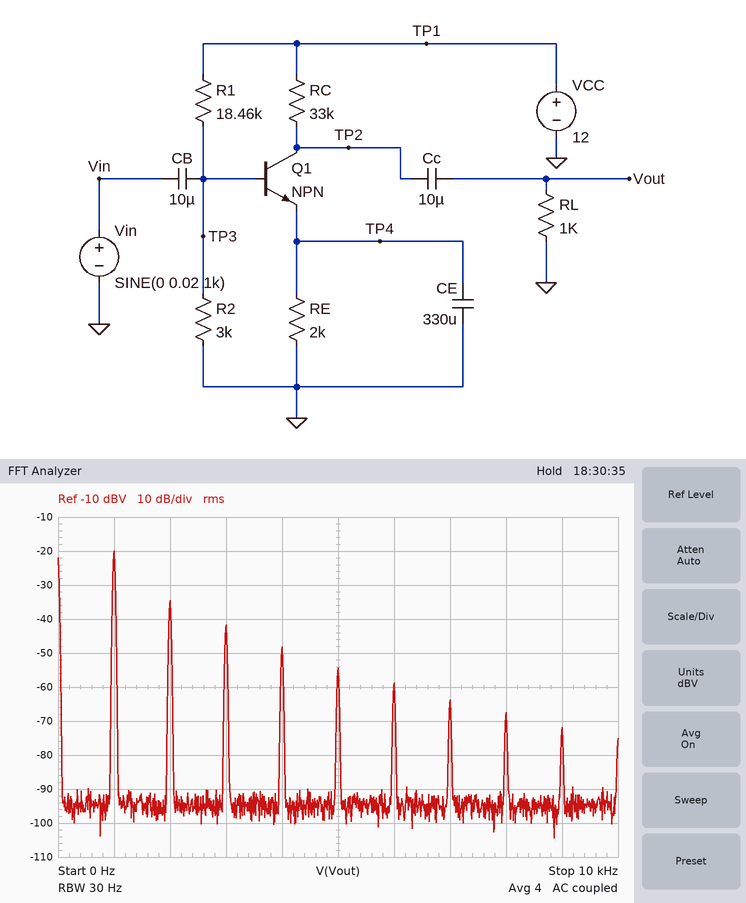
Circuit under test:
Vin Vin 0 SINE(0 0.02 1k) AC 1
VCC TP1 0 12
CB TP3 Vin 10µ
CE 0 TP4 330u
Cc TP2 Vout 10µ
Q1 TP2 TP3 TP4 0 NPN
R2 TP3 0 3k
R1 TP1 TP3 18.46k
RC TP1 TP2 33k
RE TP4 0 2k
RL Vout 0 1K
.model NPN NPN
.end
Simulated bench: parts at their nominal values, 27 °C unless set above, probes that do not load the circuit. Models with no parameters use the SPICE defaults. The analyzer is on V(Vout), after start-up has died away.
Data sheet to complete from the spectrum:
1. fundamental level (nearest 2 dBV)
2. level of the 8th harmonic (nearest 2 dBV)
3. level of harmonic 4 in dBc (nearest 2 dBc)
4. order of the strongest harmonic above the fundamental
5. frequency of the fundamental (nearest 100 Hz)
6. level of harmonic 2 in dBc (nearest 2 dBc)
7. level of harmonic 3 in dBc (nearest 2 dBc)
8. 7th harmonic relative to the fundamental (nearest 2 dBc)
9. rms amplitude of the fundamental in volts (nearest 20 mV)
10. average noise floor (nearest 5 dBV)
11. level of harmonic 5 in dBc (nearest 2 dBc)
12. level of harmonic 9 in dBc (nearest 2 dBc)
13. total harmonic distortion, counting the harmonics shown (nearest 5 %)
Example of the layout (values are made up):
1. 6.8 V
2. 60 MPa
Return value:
1. -20 dBV
2. -68 dBV
3. -28 dBc
4. 2
5. 1.0 kHz
6. -14 dBc
7. -22 dBc
8. -44 dBc
9. 100 mV
10. -95 dBV
11. -34 dBc
12. -52 dBc
13. 20 %
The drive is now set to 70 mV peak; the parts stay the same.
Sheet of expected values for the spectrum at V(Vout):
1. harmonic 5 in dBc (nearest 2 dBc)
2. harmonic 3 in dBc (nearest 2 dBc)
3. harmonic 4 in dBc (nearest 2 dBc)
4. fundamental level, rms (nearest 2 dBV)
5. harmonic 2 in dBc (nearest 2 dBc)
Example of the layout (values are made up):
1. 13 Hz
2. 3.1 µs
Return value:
1. -22 dBc
2. -34 dBc
3. -18 dBc
4. -10 dBV
5. -8 dBc
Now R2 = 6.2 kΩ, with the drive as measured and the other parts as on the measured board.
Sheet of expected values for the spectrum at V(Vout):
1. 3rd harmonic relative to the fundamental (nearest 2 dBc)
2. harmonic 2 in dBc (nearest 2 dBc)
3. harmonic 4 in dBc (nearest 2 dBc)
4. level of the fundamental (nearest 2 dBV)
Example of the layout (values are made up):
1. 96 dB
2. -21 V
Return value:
1. -20 dBc
2. -10 dBc
3. -30 dBc
4. -36 dBV
